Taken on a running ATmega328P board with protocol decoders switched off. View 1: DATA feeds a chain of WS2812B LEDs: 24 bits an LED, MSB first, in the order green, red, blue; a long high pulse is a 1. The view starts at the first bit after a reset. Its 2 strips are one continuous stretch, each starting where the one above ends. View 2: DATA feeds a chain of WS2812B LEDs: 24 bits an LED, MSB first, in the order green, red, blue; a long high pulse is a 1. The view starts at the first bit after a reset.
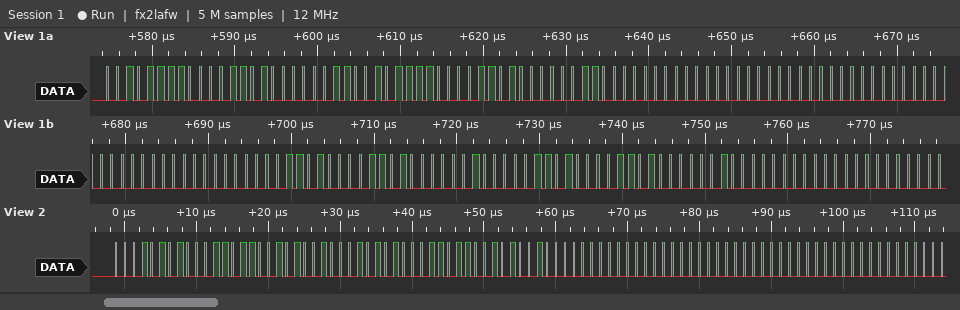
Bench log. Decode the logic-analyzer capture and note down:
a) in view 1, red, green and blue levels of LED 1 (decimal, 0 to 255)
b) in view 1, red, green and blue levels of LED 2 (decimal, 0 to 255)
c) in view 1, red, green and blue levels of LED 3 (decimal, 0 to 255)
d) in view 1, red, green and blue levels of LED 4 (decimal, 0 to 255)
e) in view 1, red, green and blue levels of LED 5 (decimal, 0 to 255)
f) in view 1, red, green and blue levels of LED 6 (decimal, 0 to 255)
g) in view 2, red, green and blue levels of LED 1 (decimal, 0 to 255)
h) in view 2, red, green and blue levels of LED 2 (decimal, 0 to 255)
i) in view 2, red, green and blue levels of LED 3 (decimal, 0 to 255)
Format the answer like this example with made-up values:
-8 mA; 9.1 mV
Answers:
13, 47, 3; 13, 47, 3; 0, 0, 0; 0, 0, 0; 13, 13, 2; 13, 13, 2; 27, 21, 41; 27, 21, 41; 0, 0, 0
